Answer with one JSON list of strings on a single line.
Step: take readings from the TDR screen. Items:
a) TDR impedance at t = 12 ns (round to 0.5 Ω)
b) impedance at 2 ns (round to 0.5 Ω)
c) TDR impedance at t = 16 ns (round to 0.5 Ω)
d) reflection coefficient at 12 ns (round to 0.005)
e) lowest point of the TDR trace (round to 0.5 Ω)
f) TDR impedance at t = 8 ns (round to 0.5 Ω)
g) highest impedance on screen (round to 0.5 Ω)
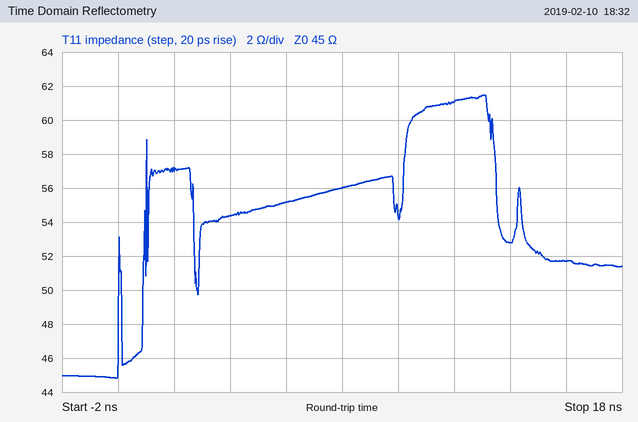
["61.0 Ω", "57.0 Ω", "51.5 Ω", "+0.150", "45.0 Ω", "56.0 Ω", "61.5 Ω"]
